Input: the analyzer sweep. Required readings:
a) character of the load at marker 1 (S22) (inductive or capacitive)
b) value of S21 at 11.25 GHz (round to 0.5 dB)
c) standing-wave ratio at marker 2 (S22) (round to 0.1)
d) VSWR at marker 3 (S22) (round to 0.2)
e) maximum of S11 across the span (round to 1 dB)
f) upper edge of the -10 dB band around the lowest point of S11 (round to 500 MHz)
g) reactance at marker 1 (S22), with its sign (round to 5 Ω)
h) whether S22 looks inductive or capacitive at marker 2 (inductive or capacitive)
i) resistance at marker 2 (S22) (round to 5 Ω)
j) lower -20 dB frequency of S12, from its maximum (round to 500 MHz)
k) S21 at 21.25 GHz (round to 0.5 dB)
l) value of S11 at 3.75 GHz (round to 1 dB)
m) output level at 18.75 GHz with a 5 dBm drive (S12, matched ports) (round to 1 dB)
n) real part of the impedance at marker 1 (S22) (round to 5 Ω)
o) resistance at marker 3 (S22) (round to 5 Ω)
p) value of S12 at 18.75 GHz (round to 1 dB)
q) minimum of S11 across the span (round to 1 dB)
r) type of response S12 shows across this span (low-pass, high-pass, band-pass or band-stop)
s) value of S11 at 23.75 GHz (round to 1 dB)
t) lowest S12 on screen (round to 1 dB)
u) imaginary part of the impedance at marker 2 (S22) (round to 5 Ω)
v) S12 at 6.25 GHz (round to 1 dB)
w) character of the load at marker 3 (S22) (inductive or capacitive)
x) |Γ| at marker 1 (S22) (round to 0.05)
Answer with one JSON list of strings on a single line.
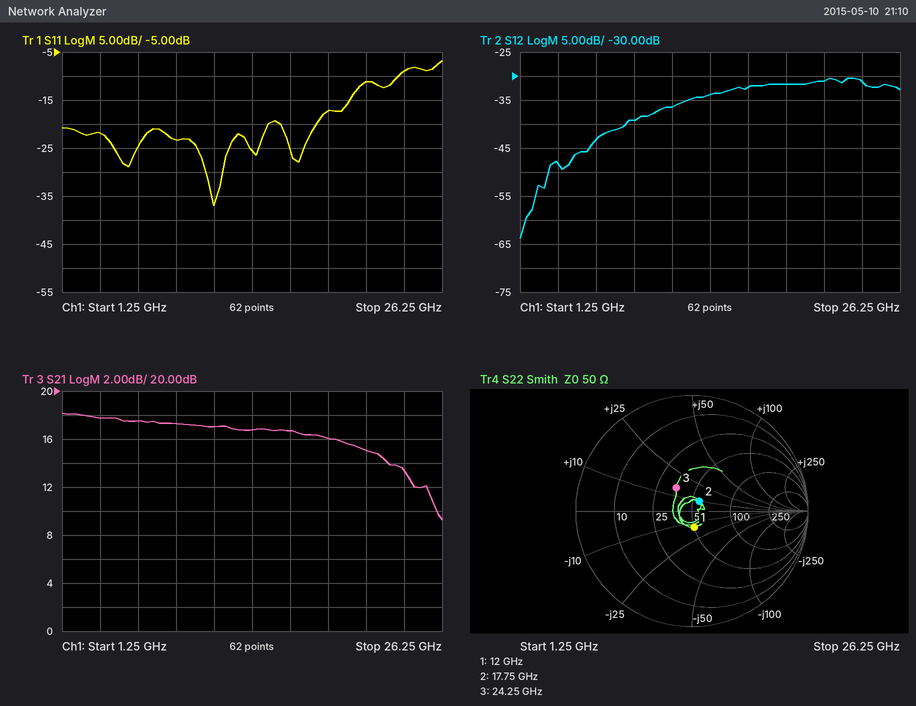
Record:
["capacitive", "17.0 dB", "1.2", "1.6", "-7 dB", "23.5 GHz", "-15 Ω", "inductive", "55 Ω", "3.0 GHz", "15.0 dB", "-22 dB", "-27 dBm", "50 Ω", "35 Ω", "-32 dB", "-37 dB", "high-pass", "-9 dB", "-64 dB", "+10 Ω", "-43 dB", "inductive", "0.15"]
